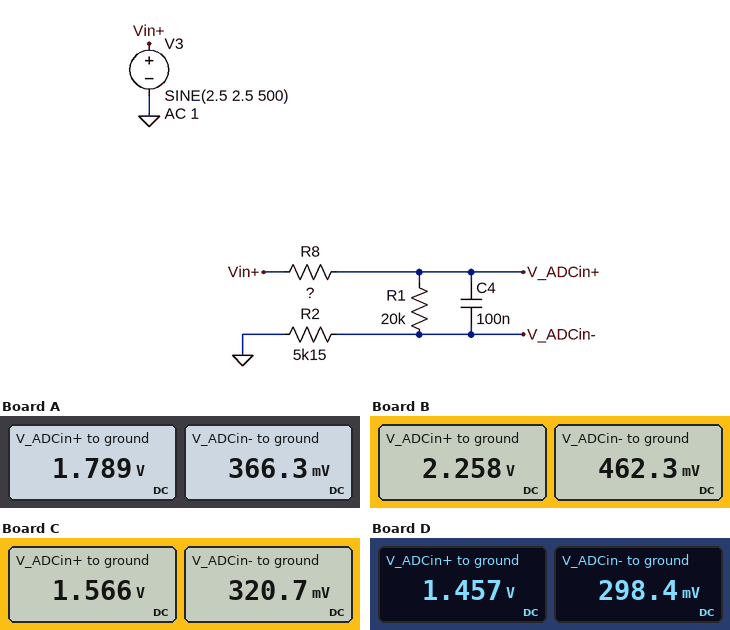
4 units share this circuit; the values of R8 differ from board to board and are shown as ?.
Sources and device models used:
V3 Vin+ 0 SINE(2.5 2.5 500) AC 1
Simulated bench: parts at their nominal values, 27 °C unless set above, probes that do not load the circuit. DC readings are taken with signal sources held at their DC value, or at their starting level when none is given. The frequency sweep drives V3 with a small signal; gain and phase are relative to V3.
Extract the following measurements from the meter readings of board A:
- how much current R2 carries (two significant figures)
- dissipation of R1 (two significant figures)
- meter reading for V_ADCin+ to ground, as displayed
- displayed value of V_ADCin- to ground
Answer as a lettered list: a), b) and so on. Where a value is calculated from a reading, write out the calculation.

a) (366.3 mV) / 5.15 kΩ = 71 µA
b) (1.789 V - 366.3 mV)^2 / 20 kΩ = 100 µW
c) 1.789 V
d) 366.3 mV
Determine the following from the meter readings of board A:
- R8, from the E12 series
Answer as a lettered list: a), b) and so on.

a) 10 kΩ
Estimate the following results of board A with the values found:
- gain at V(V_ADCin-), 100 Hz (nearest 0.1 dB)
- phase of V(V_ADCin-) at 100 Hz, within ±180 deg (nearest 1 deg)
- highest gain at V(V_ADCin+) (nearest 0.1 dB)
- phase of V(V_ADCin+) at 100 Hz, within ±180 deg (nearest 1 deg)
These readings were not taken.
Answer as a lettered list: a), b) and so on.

a) -13.7 dB
b) 23 deg
c) -2.9 dB
d) -14 deg
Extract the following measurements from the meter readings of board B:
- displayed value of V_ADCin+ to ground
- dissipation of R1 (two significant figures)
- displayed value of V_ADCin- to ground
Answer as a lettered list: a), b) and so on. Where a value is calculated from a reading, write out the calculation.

a) 2.258 V
b) (2.258 V - 462.3 mV)^2 / 20 kΩ = 160 µW
c) 462.3 mV
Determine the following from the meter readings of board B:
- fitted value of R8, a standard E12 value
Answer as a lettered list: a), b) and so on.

a) 2.7 kΩ
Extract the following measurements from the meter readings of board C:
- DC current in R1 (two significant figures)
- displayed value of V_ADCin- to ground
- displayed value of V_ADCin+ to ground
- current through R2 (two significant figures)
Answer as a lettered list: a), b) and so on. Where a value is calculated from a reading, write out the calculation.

a) (1.566 V - 320.7 mV) / 20 kΩ = 62 µA
b) 320.7 mV
c) 1.566 V
d) (320.7 mV) / 5.15 kΩ = 62 µA
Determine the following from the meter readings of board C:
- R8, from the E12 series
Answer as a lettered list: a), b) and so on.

a) 15 kΩ
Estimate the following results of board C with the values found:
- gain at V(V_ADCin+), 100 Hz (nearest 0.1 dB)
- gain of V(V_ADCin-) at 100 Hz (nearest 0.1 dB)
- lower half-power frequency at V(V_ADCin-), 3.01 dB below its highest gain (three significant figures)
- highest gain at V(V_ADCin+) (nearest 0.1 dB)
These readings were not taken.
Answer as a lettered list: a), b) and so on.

a) -5.2 dB
b) -15.2 dB
c) 112 Hz
d) -4.1 dB
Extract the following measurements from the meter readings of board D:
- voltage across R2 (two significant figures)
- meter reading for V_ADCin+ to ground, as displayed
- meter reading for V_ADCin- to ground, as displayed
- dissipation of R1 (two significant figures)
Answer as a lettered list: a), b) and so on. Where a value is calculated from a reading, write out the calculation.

a) 298.4 mV = 300 mV
b) 1.457 V
c) 298.4 mV
d) (1.457 V - 298.4 mV)^2 / 20 kΩ = 67 µW
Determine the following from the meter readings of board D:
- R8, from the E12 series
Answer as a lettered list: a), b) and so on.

a) 18 kΩ
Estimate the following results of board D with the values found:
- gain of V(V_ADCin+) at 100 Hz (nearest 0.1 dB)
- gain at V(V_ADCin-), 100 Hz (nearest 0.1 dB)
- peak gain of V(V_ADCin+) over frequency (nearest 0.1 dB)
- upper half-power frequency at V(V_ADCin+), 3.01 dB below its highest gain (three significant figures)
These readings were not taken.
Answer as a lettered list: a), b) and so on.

a) -6.0 dB
b) -16.0 dB
c) -4.7 dB
d) 176 Hz
